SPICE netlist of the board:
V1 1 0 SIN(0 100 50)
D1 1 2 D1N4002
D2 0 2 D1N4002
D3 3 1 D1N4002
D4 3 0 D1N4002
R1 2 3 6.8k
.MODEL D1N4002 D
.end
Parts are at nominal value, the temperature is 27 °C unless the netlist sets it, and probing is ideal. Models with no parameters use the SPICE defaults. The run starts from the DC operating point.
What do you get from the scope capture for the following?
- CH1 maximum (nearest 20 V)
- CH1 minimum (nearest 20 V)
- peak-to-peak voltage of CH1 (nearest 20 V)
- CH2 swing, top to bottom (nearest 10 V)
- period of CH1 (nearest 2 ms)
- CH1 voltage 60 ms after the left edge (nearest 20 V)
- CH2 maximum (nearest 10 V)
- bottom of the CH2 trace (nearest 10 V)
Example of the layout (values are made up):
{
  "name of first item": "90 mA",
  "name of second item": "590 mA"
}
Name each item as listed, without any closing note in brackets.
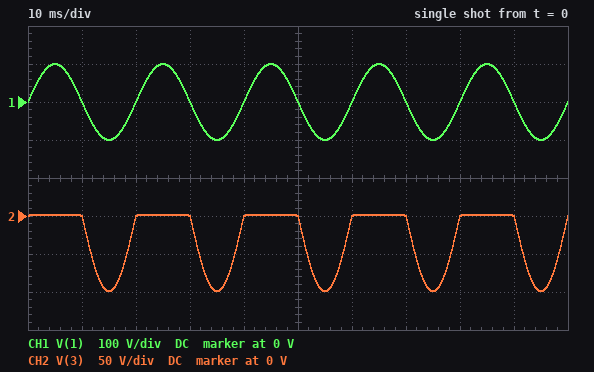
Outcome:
{
  "CH1 maximum": "100 V",
  "CH1 minimum": "-100 V",
  "peak-to-peak voltage of CH1": "200 V",
  "CH2 swing, top to bottom": "100 V",
  "period of CH1": "20 ms",
  "CH1 voltage 60 ms after the left edge": "0 V",
  "CH2 maximum": "0 V",
  "bottom of the CH2 trace": "-100 V"
}
